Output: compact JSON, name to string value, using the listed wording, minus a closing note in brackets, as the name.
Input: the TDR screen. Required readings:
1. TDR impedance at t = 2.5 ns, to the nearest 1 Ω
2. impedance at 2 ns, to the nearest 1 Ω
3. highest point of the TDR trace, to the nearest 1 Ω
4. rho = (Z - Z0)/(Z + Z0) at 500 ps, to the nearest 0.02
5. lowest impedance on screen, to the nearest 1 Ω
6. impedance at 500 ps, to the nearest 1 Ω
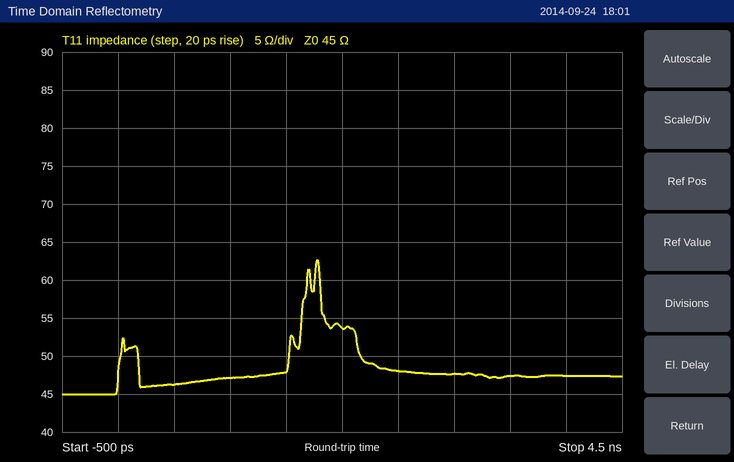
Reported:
{"TDR impedance at t = 2.5 ns, to the nearest 1 Ω": "48 Ω", "impedance at 2 ns, to the nearest 1 Ω": "54 Ω", "highest point of the TDR trace, to the nearest 1 Ω": "63 Ω", "rho = (Z - Z0)/(Z + Z0) at 500 ps, to the nearest 0.02": "+0.02", "lowest impedance on screen, to the nearest 1 Ω": "45 Ω", "impedance at 500 ps, to the nearest 1 Ω": "46 Ω"}
